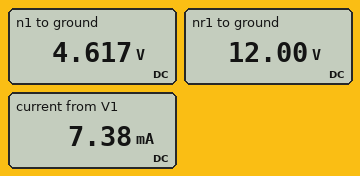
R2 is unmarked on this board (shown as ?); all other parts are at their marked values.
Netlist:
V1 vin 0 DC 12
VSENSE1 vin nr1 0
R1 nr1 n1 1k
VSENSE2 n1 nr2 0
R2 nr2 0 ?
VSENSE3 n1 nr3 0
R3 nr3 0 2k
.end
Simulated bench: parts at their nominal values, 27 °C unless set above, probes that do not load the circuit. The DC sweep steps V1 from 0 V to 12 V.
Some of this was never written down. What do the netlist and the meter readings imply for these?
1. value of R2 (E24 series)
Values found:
910 Ω
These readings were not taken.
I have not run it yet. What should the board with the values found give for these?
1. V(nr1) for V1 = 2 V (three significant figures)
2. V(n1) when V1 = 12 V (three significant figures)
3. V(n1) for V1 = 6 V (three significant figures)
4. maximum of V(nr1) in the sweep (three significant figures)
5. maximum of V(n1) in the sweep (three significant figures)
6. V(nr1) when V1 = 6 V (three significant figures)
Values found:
2.00 V
4.62 V
2.31 V
12.0 V
4.62 V
6.00 V
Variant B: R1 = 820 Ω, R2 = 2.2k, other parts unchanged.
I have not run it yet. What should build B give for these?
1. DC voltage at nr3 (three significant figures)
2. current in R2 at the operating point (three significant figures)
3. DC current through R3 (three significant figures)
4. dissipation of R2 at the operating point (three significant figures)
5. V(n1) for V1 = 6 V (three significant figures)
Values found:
6.73 V
3.06 mA
3.37 mA
20.6 mW
3.37 V
